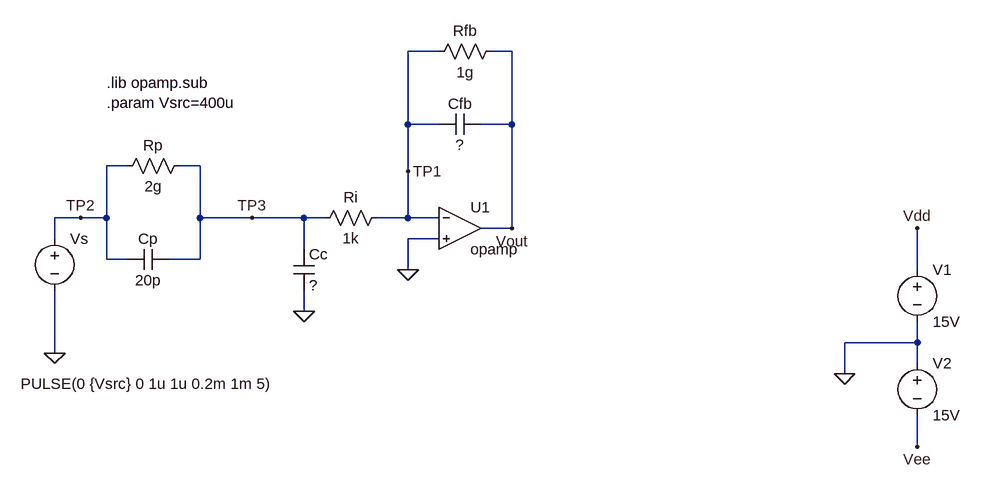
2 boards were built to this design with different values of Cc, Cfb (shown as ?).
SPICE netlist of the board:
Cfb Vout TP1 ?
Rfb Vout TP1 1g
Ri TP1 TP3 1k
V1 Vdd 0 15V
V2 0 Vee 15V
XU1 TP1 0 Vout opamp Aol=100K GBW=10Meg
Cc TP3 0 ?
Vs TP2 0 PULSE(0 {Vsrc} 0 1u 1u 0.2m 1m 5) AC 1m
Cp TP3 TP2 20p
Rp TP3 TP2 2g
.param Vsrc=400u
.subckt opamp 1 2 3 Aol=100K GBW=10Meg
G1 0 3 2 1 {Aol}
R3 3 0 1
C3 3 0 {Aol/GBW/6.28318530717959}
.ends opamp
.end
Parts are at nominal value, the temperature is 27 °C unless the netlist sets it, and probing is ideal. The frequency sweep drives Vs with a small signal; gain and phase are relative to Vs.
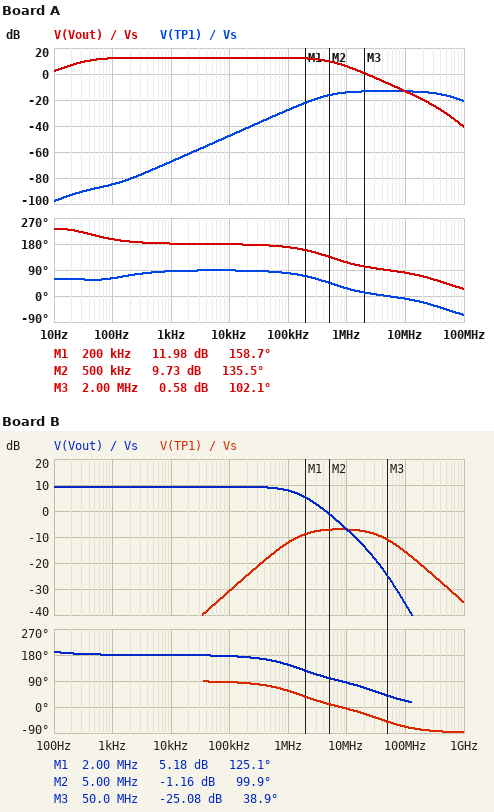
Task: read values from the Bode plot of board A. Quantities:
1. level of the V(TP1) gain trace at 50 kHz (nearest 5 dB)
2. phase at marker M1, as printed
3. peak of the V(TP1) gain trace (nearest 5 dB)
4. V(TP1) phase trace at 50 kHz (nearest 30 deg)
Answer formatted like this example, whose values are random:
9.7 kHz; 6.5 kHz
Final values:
-35 dB; 158.7 deg; -15 dB; 90 deg
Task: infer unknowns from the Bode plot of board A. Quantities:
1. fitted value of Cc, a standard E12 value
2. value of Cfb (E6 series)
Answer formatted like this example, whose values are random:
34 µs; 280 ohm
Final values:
47 pF; 4.7 pF
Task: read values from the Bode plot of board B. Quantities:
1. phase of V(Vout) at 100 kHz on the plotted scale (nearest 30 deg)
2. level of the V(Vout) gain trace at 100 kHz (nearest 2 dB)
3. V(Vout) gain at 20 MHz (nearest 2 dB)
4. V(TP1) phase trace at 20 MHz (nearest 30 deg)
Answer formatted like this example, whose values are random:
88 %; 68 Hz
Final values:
180 deg; 10 dB; -14 dB; -30 deg
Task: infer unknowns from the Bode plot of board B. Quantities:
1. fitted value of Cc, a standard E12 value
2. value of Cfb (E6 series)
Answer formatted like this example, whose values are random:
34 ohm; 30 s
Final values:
6.8 pF; 6.8 pF
